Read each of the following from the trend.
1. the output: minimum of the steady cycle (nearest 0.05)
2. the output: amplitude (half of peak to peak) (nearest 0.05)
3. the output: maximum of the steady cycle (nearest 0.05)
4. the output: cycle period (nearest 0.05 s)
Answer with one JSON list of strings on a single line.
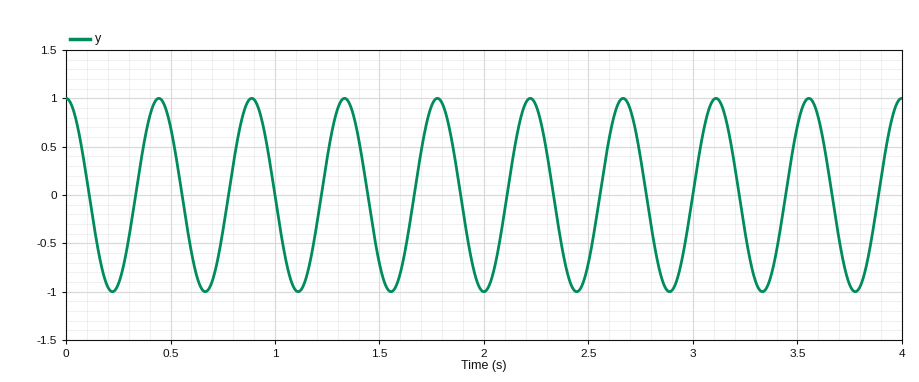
["-1.00", "1.00", "1.00", "0.45 s"]
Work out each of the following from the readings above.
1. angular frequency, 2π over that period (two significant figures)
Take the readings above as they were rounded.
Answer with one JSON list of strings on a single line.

["14 rad/s"]
